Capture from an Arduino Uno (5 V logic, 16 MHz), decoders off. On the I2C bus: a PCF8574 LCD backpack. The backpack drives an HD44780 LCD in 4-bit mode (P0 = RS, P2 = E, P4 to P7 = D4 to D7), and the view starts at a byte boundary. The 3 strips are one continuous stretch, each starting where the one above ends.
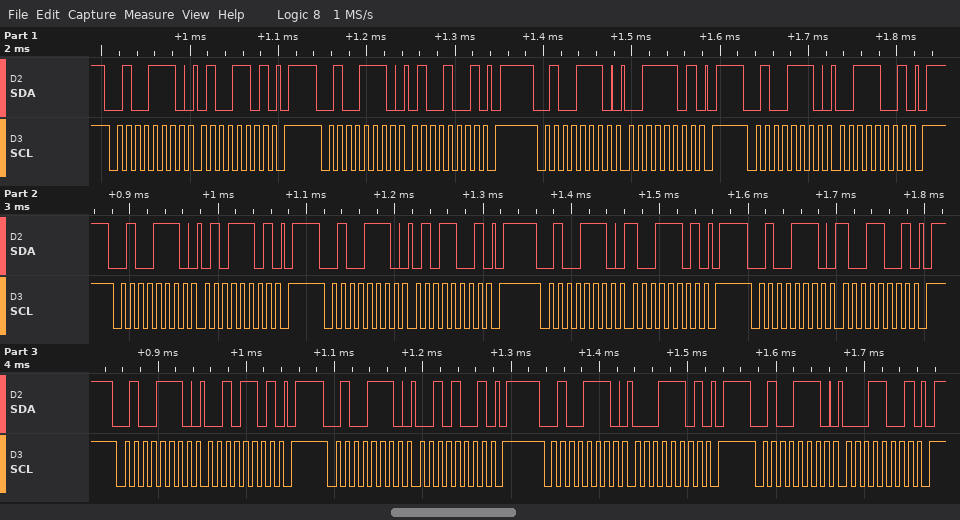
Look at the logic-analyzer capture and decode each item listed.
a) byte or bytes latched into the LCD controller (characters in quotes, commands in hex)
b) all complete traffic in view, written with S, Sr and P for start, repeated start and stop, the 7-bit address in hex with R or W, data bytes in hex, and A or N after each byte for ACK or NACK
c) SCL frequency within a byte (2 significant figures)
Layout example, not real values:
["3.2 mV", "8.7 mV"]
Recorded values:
["'C' 'Y' '!'", "S 27W A 4D A P S 27W A 49 A P S 27W A 3D A P S 27W A 39 A P S 27W A 5D A P S 27W A 59 A P S 27W A 9D A P S 27W A 99 A P S 27W A 2D A P S 27W A 29 A P S 27W A 1D A P S 27W A 19 A P", "100 kHz"]
